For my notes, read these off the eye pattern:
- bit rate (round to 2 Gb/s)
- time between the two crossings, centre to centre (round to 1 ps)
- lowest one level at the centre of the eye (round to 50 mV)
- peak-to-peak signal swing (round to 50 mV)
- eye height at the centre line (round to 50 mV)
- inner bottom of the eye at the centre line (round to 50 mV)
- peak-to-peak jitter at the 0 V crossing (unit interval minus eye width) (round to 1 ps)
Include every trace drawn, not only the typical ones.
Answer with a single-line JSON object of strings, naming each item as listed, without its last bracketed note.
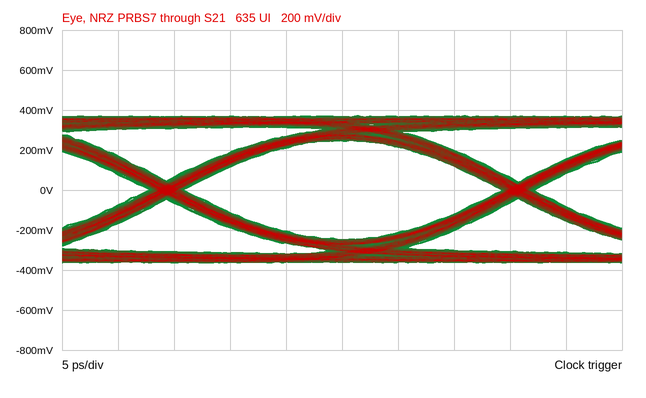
{"bit rate": "32 Gb/s", "time between the two crossings, centre to centre": "31 ps", "lowest one level at the centre of the eye": "250 mV", "peak-to-peak signal swing": "750 mV", "eye height at the centre line": "500 mV", "inner bottom of the eye at the centre line": "-250 mV", "peak-to-peak jitter at the 0 V crossing (unit interval minus eye width)": "3 ps"}
